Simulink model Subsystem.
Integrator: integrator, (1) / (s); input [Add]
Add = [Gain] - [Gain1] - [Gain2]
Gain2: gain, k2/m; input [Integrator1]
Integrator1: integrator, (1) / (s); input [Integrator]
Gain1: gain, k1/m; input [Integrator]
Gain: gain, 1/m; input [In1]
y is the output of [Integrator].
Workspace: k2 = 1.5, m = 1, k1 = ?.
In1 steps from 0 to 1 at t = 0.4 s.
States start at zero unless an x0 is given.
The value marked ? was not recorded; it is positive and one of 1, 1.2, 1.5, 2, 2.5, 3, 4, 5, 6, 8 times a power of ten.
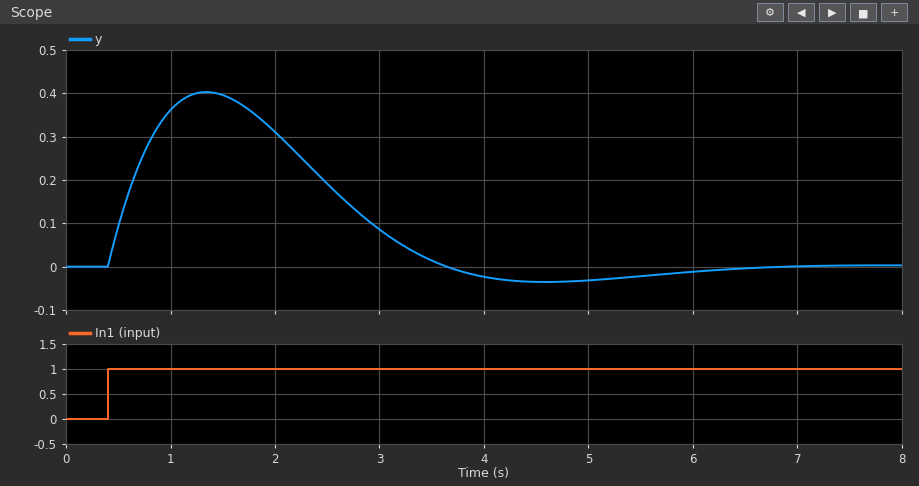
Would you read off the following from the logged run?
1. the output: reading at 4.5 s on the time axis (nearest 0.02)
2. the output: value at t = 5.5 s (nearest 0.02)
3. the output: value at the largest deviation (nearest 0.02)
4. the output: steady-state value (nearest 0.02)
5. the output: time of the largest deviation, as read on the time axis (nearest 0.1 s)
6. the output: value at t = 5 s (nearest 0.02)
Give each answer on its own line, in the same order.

-0.04
-0.02
0.40
0.00
1.3 s
-0.04
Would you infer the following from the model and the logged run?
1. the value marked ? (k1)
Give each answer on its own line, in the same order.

1.5
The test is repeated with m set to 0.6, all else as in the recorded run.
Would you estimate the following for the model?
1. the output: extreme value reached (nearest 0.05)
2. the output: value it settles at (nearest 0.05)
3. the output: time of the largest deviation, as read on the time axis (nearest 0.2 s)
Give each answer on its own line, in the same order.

0.45
0.00
1.0 s
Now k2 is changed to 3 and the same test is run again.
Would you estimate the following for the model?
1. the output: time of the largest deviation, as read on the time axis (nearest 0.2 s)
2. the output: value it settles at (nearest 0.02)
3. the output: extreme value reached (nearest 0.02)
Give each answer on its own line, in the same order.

1.2 s
0.00
0.34
